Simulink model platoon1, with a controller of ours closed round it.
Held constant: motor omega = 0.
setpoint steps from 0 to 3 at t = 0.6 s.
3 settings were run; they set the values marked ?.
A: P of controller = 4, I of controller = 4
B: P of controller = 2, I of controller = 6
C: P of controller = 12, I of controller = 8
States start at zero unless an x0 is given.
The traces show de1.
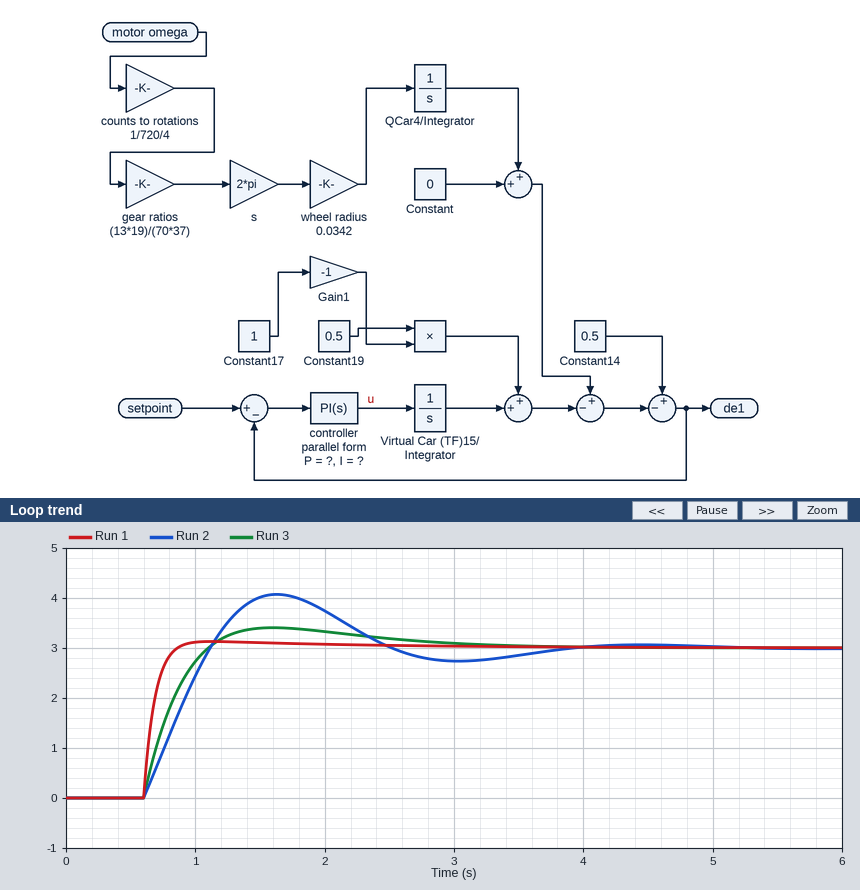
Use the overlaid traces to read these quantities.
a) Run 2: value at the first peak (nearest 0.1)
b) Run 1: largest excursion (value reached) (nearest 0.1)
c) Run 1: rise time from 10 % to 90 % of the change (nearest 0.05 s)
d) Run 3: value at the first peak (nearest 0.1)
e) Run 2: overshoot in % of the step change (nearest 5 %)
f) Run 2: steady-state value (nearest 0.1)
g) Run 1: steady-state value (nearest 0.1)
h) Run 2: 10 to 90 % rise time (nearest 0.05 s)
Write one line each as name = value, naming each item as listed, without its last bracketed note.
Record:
Run 2: value at the first peak = 4.1
Run 1: largest excursion (value reached) = 3.1
Run 1: rise time from 10 % to 90 % of the change = 0.15 s
Run 3: value at the first peak = 3.4
Run 2: overshoot in % of the step change = 35 %
Run 2: steady-state value = 3.0
Run 1: steady-state value = 3.0
Run 2: 10 to 90 % rise time = 0.40 s
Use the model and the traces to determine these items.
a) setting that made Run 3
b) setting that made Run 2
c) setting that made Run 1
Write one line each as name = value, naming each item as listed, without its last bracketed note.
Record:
setting that made Run 3 = A
setting that made Run 2 = B
setting that made Run 1 = C
